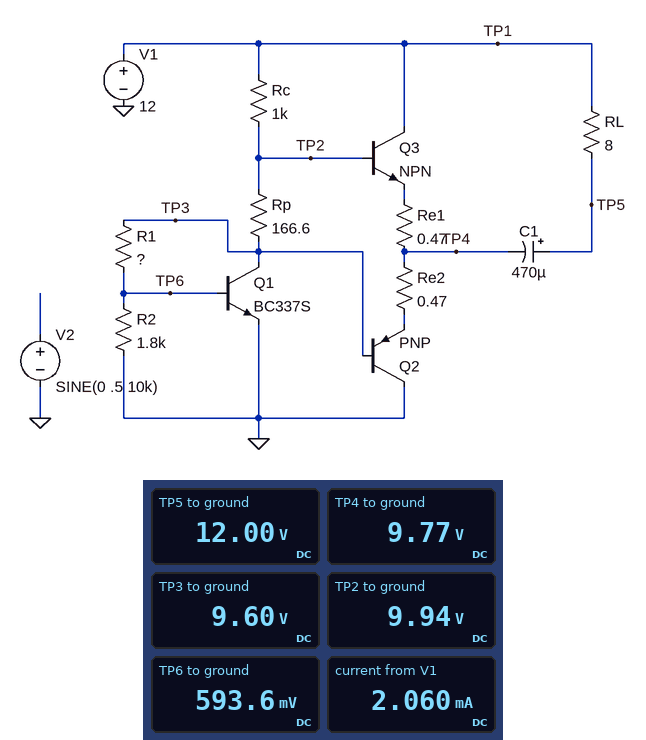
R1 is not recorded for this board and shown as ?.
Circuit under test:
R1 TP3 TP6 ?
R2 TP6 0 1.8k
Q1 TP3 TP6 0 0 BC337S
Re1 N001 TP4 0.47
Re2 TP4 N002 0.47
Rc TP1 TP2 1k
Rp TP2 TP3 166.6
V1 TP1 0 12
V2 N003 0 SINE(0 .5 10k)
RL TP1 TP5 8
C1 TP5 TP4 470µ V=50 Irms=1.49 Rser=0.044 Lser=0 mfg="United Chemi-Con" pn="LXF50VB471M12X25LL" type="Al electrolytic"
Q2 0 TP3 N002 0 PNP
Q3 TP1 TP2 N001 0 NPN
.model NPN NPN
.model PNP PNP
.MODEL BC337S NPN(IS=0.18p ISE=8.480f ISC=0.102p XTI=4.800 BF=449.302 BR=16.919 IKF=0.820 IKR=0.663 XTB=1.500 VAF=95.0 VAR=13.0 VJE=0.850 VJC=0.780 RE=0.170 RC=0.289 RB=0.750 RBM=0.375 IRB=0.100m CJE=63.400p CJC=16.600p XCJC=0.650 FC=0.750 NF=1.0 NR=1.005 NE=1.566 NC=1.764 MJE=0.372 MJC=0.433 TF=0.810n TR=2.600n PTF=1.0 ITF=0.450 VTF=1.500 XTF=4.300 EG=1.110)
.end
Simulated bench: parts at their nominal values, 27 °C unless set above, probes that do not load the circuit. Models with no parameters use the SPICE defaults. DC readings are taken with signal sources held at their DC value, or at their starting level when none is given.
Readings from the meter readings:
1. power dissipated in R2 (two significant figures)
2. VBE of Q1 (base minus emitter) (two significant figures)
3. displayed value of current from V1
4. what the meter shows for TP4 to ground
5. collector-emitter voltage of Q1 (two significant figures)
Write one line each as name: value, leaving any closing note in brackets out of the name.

power dissipated in R2: 200 µW
VBE of Q1 (base minus emitter): 590 mV
displayed value of current from V1: 2.060 mA
what the meter shows for TP4 to ground: 9.77 V
collector-emitter voltage of Q1: 9.6 V
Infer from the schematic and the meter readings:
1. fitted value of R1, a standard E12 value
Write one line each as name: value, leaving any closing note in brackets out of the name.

fitted value of R1, a standard E12 value: 27 kΩ
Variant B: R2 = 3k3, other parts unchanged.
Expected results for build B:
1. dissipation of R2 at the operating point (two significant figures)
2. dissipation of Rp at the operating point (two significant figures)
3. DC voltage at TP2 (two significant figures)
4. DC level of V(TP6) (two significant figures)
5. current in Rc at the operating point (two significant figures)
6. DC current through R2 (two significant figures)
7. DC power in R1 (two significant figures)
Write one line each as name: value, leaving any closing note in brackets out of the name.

dissipation of R2 at the operating point: 120 µW
dissipation of Rp at the operating point: 4.4 mW
DC voltage at TP2: 6.9 V
DC level of V(TP6): 620 mV
current in Rc at the operating point: 5.1 mA
DC current through R2: 190 µA
DC power in R1: 1.1 mW
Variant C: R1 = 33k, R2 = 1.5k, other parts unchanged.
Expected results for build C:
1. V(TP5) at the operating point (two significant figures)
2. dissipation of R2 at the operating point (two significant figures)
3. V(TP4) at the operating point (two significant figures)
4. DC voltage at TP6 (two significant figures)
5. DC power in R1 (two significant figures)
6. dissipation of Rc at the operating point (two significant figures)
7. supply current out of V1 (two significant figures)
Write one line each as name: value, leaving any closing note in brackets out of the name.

V(TP5) at the operating point: 12 V
dissipation of R2 at the operating point: 170 µW
V(TP4) at the operating point: 12 V
DC voltage at TP6: 500 mV
DC power in R1: 3.7 mW
dissipation of Rc at the operating point: 150 µW
supply current out of V1: 390 µA
